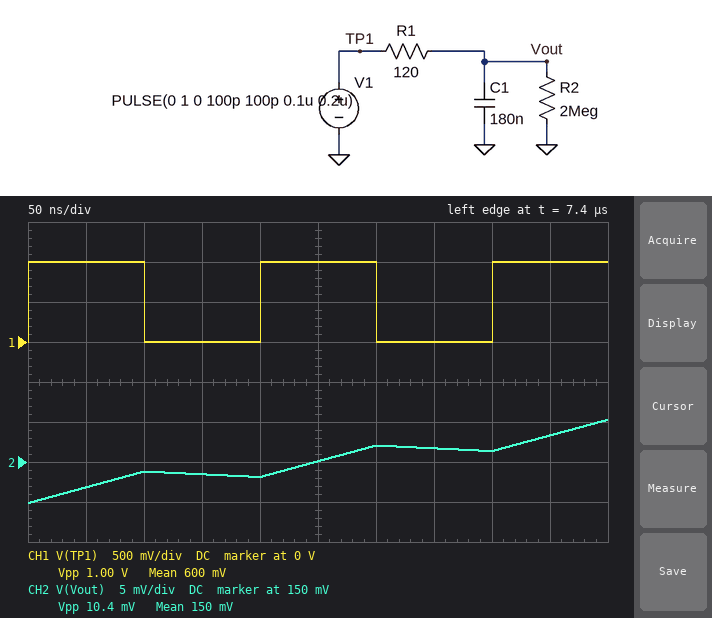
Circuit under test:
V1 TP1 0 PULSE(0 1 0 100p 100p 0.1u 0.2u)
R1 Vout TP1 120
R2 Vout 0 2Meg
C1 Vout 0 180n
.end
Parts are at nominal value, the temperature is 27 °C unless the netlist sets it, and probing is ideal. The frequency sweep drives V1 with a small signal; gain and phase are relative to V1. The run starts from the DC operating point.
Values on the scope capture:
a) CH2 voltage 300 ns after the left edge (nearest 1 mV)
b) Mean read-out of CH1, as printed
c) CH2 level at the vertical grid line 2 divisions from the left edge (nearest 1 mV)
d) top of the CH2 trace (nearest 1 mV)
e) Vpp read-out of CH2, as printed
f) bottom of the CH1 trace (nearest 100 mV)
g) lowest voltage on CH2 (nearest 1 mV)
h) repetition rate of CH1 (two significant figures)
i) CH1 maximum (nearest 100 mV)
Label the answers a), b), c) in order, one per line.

a) 152 mV
b) 600 mV
c) 149 mV
d) 155 mV
e) 10.4 mV
f) 0 V
g) 145 mV
h) 5.0 MHz
i) 1.0 V
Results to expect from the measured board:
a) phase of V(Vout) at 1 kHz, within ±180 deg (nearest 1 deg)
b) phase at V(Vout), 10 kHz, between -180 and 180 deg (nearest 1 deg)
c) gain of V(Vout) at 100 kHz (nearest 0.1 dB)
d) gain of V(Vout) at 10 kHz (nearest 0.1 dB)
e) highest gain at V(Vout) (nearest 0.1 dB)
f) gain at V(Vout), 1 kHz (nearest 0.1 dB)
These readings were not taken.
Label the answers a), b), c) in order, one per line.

a) -8 deg
b) -54 deg
c) -22.7 dB
d) -4.5 dB
e) 0 dB
f) -0.1 dB
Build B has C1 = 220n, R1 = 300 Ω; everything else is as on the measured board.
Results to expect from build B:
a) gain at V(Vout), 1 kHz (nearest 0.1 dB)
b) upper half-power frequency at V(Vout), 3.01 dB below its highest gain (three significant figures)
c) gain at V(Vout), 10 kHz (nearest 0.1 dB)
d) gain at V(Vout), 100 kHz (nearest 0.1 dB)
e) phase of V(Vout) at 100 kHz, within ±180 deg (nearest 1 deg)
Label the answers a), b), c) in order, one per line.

a) -0.7 dB
b) 2.41 kHz
c) -12.6 dB
d) -32.4 dB
e) -89 deg
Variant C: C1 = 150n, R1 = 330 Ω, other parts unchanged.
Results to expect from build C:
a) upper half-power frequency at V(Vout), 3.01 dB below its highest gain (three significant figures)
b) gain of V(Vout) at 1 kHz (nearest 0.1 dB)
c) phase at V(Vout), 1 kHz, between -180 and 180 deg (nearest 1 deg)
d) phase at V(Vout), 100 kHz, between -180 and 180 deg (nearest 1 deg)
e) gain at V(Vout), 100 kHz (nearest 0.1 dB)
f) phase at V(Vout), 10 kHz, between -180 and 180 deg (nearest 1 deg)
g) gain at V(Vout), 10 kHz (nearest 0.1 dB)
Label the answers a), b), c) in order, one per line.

a) 3.22 kHz
b) -0.4 dB
c) -17 deg
d) -88 deg
e) -29.9 dB
f) -72 deg
g) -10.3 dB
